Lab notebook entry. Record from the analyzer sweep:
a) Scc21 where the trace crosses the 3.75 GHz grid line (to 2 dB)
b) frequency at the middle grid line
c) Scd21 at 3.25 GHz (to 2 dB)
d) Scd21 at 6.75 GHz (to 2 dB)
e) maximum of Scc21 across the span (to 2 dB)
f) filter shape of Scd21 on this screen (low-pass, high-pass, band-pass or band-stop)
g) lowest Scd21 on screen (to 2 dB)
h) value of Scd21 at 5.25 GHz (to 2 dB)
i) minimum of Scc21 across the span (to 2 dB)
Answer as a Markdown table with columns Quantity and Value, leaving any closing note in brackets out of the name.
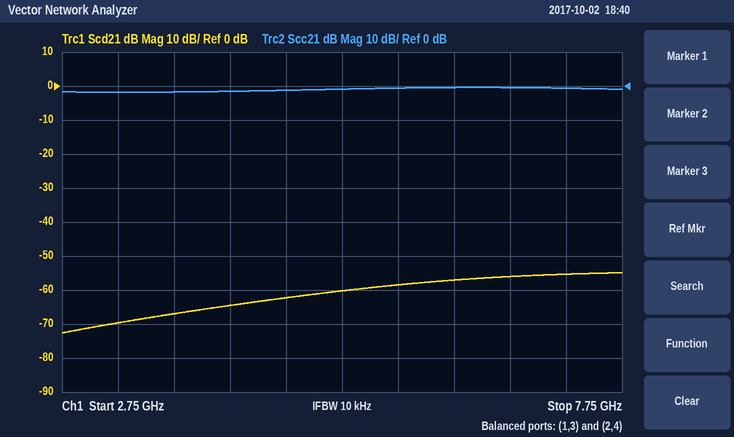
| Quantity | Value |
|---|---|
| Scc21 where the trace crosses the 3.75 GHz grid line | -2 dB |
| frequency at the middle grid line | 5.25 GHz |
| Scd21 at 3.25 GHz | -70 dB |
| Scd21 at 6.75 GHz | -56 dB |
| maximum of Scc21 across the span | 0 dB |
| filter shape of Scd21 on this screen | high-pass |
| lowest Scd21 on screen | -72 dB |
| value of Scd21 at 5.25 GHz | -60 dB |
| minimum of Scc21 across the span | -2 dB |
